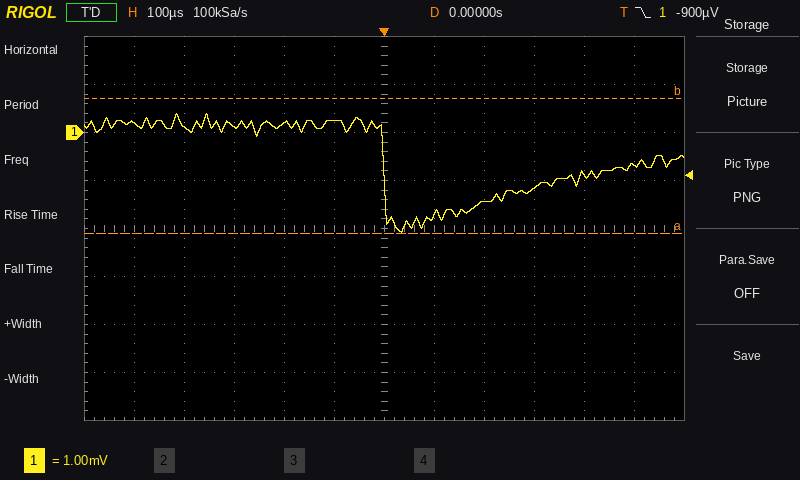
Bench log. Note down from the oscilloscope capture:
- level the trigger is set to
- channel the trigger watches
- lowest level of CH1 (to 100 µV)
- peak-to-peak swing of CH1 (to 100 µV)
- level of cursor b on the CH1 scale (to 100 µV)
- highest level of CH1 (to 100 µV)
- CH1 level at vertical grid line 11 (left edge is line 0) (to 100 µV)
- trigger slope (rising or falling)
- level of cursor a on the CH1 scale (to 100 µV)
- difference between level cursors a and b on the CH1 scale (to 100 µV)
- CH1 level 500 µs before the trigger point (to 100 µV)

-900 µV
CH1
-2.1 mV
2.5 mV
700 µV
400 µV
-700 µV
falling
-2.1 mV
2.8 mV
200 µV
